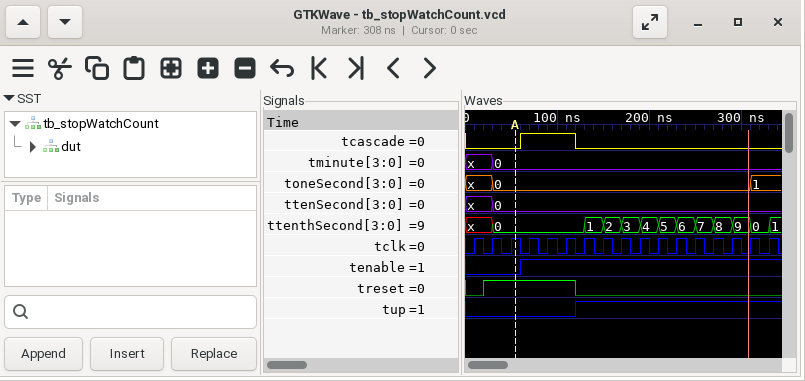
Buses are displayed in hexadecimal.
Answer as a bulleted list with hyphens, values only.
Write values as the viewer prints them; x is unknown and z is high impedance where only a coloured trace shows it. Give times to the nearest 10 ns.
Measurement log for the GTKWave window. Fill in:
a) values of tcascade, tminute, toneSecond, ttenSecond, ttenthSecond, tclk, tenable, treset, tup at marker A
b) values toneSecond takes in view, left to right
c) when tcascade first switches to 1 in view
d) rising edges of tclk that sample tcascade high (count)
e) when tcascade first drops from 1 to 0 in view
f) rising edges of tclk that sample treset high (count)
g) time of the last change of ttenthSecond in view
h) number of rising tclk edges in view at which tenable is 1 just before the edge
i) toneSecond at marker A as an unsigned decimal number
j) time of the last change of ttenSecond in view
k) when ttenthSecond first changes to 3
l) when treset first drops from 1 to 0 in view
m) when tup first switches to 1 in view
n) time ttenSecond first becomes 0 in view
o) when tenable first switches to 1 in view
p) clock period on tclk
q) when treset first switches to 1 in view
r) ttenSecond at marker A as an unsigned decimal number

- tcascade=0, tminute=0, toneSecond=0, ttenSecond=0, ttenthSecond=0, tclk=1, tenable=0, treset=1, tup=0
- x, 0, 1
- 60 ns
- 3
- 120 ns
- 5
- 330 ns
- 14
- 0
- 30 ns
- 170 ns
- 120 ns
- 120 ns
- 30 ns
- 60 ns
- 20 ns
- 20 ns
- 0
